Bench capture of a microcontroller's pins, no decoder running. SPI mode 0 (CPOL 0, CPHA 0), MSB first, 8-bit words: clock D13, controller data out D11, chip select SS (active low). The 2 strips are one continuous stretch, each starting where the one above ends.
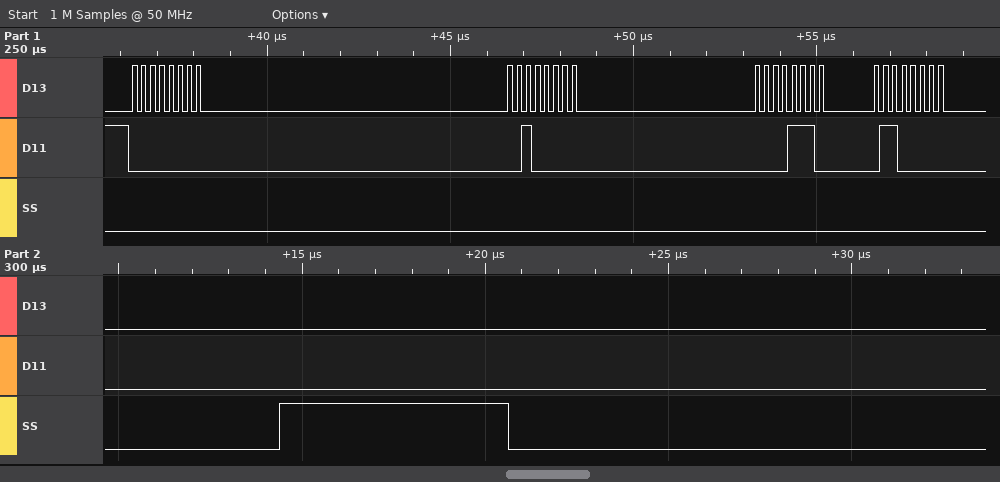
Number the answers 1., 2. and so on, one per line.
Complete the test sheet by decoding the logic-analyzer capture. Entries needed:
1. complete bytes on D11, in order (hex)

1. 0x00 0x20 0x0E 0x60
